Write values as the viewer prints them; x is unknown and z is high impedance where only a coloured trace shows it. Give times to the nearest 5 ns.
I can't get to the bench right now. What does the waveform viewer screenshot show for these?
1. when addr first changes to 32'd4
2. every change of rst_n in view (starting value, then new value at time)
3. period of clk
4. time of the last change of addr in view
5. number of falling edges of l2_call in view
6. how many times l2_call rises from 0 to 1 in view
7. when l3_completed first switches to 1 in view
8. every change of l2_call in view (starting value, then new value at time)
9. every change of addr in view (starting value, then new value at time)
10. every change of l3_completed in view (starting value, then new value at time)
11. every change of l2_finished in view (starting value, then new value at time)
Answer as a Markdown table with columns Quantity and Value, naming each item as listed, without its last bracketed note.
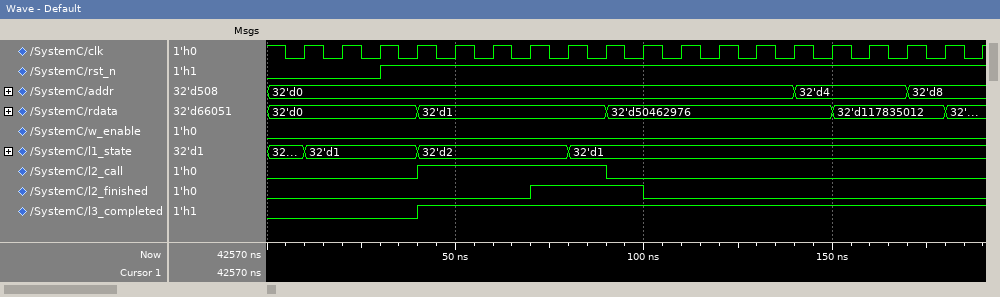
| Quantity | Value |
|---|---|
| when addr first changes to 32'd4 | 140 ns |
| every change of rst_n in view | 0, 1 at 30 ns |
| period of clk | 10 ns |
| time of the last change of addr in view | 170 ns |
| number of falling edges of l2_call in view | 1 |
| how many times l2_call rises from 0 to 1 in view | 1 |
| when l3_completed first switches to 1 in view | 40 ns |
| every change of l2_call in view | 0, 1 at 40 ns, 0 at 90 ns |
| every change of addr in view | 32'd0, 32'd4 at 140 ns, 32'd8 at 170 ns |
| every change of l3_completed in view | 0, 1 at 40 ns |
| every change of l2_finished in view | 0, 1 at 70 ns, 0 at 100 ns |
